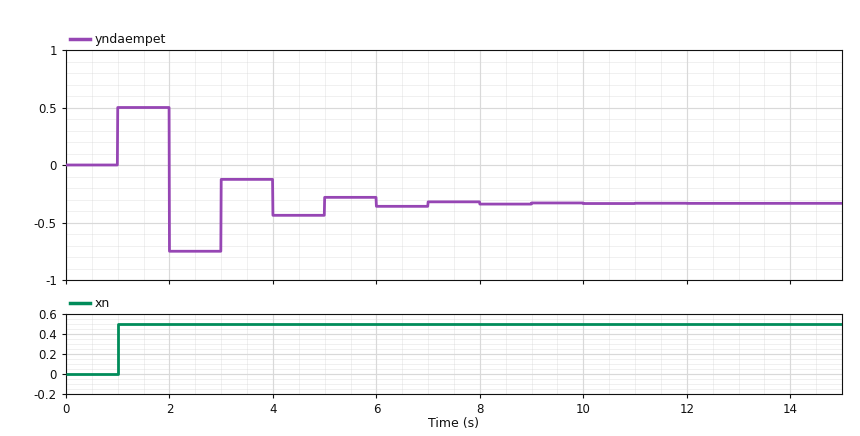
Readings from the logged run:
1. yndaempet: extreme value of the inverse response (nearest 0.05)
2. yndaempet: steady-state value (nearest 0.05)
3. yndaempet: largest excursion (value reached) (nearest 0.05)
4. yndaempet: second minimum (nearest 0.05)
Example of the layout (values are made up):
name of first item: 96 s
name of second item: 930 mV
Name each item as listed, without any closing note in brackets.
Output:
yndaempet: extreme value of the inverse response: 0.50
yndaempet: steady-state value: -0.35
yndaempet: largest excursion (value reached): -0.75
yndaempet: second minimum: -0.45
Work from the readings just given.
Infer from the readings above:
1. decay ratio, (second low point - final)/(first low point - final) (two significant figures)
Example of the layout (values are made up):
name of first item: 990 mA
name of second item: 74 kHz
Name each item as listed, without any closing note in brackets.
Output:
decay ratio, (second low point - final)/(first low point - final): 0.25
